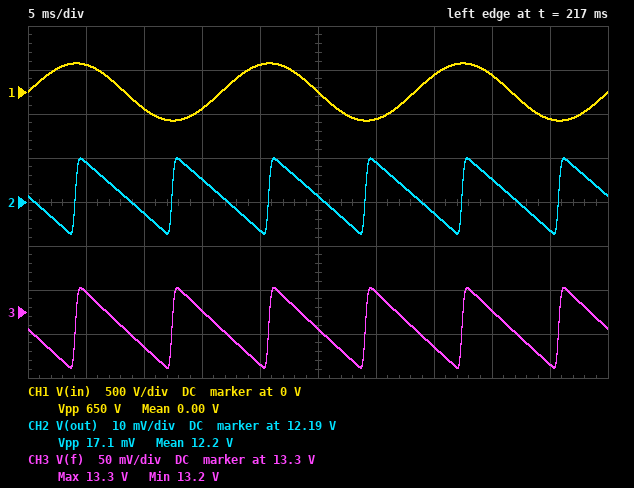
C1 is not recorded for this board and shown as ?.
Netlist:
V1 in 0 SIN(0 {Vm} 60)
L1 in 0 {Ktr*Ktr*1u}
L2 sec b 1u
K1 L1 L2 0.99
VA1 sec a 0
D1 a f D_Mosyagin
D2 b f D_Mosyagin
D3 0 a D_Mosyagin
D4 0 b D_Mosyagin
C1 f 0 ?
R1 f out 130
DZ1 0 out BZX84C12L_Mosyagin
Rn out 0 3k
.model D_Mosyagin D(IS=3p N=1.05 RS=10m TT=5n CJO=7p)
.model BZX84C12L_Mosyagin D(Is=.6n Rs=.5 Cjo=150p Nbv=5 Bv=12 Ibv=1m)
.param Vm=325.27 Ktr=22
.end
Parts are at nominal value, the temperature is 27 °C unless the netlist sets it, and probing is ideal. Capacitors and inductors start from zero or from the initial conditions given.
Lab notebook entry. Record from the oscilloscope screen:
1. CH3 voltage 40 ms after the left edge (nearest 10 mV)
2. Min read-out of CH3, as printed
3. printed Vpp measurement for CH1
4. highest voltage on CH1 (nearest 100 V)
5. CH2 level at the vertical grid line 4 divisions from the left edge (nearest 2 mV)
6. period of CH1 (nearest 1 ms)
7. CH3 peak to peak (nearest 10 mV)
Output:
13.30 V
13.2 V
650 V
300 V
12.184 V
17 ms
90 mV
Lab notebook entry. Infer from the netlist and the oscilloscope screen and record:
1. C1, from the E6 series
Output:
680 µF
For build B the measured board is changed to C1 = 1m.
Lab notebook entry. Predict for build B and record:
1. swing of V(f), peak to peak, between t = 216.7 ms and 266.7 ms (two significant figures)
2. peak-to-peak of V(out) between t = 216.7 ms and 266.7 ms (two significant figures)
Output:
62 mV
12 mV
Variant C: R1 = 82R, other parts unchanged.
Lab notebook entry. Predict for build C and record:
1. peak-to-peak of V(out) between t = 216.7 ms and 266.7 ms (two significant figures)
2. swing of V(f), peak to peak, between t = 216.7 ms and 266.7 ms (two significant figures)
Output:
22 mV
130 mV
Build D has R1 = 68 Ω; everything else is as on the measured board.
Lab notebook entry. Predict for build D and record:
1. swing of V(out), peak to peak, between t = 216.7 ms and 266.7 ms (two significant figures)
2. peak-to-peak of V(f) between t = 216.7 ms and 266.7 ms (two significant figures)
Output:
25 mV
150 mV
